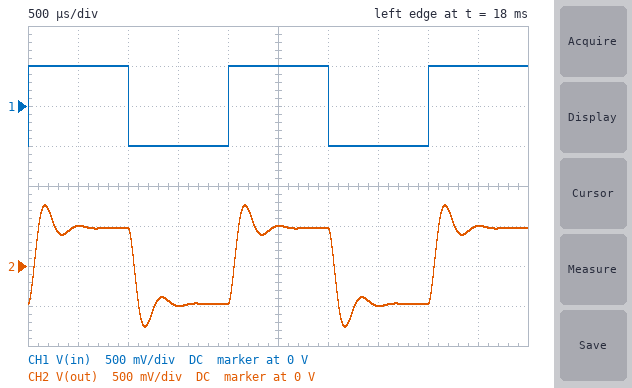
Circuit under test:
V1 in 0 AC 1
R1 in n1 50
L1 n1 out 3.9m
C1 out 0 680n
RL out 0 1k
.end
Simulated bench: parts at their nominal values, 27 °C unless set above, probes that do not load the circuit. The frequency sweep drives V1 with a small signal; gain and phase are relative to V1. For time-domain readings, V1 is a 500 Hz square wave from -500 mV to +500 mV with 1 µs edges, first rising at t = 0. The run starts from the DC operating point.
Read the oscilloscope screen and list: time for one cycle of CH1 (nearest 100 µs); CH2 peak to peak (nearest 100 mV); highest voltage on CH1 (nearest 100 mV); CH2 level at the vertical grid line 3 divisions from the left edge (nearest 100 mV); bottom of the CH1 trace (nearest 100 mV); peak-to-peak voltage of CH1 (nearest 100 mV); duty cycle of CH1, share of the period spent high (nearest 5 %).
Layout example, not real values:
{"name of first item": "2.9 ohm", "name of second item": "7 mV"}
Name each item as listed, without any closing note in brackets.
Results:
{"time for one cycle of CH1": "2.0 ms", "CH2 peak to peak": "1.5 V", "highest voltage on CH1": "500 mV", "CH2 level at the vertical grid line 3 divisions from the left edge": "-500 mV", "bottom of the CH1 trace": "-500 mV", "peak-to-peak voltage of CH1": "1.0 V", "duty cycle of CH1, share of the period spent high": "50 %"}
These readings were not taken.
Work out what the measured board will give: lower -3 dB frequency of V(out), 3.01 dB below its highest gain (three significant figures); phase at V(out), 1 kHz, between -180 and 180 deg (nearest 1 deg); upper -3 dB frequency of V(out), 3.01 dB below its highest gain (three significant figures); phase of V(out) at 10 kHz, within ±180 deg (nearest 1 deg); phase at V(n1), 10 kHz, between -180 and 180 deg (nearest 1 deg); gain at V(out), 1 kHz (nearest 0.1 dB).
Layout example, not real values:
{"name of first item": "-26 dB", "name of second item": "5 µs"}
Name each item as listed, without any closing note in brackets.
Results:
{"lower -3 dB frequency of V(out), 3.01 dB below its highest gain": "848 Hz", "phase at V(out), 1 kHz, between -180 and 180 deg": "-14 deg", "upper -3 dB frequency of V(out), 3.01 dB below its highest gain": "3.76 kHz", "phase of V(out) at 10 kHz, within ±180 deg": "-166 deg", "phase at V(n1), 10 kHz, between -180 and 180 deg": "13 deg", "gain at V(out), 1 kHz": "0.2 dB"}
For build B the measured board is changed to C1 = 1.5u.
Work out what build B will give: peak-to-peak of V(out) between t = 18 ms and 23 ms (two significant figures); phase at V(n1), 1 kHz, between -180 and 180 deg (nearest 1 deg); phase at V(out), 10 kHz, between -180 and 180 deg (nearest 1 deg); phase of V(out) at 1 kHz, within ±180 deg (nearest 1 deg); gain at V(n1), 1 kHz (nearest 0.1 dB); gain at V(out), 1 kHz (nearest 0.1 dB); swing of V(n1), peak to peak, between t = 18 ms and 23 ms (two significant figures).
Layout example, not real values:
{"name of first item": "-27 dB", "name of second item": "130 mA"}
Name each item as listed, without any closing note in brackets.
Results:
{"peak-to-peak of V(out) between t = 18 ms and 23 ms": "1.3 V", "phase at V(n1), 1 kHz, between -180 and 180 deg": "-29 deg", "phase at V(out), 10 kHz, between -180 and 180 deg": "-167 deg", "phase of V(out) at 1 kHz, within ±180 deg": "-31 deg", "gain at V(n1), 1 kHz": "-1.9 dB", "gain at V(out), 1 kHz": "0.4 dB", "swing of V(n1), peak to peak, between t = 18 ms and 23 ms": "1.1 V"}
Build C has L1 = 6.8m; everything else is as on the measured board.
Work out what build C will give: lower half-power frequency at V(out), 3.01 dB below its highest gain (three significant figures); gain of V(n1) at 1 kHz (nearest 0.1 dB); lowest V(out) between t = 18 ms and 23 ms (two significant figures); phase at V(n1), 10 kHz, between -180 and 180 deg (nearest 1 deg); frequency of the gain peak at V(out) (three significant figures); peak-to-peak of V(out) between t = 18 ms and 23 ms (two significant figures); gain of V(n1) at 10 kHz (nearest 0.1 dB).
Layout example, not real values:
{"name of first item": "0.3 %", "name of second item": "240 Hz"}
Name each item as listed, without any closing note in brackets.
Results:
{"lower half-power frequency at V(out), 3.01 dB below its highest gain": "1.24 kHz", "gain of V(n1) at 1 kHz": "-0.9 dB", "lowest V(out) between t = 18 ms and 23 ms": "-840 mV", "phase at V(n1), 10 kHz, between -180 and 180 deg": "7 deg", "frequency of the gain peak at V(out)": "2.18 kHz", "peak-to-peak of V(out) between t = 18 ms and 23 ms": "1.7 V", "gain of V(n1) at 10 kHz": "-0.1 dB"}
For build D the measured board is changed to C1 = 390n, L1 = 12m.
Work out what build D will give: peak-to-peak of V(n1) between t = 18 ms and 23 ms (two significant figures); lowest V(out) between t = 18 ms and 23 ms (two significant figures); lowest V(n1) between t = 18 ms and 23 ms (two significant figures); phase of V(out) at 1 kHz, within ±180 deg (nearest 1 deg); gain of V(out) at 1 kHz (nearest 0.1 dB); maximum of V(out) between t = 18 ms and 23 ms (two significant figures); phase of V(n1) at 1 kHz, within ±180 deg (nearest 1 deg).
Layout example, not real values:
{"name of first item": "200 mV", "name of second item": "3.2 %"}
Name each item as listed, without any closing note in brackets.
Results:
{"peak-to-peak of V(n1) between t = 18 ms and 23 ms": "1.1 V", "lowest V(out) between t = 18 ms and 23 ms": "-940 mV", "lowest V(n1) between t = 18 ms and 23 ms": "-570 mV", "phase of V(out) at 1 kHz, within ±180 deg": "-13 deg", "gain of V(out) at 1 kHz": "1.0 dB", "maximum of V(out) between t = 18 ms and 23 ms": "940 mV", "phase of V(n1) at 1 kHz, within ±180 deg": "-8 deg"}
